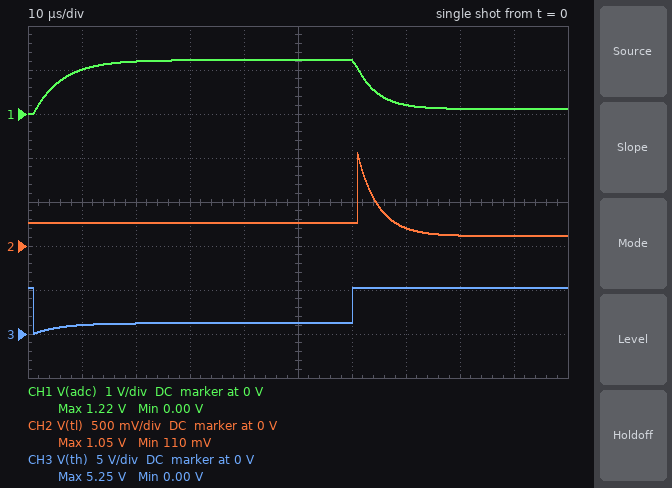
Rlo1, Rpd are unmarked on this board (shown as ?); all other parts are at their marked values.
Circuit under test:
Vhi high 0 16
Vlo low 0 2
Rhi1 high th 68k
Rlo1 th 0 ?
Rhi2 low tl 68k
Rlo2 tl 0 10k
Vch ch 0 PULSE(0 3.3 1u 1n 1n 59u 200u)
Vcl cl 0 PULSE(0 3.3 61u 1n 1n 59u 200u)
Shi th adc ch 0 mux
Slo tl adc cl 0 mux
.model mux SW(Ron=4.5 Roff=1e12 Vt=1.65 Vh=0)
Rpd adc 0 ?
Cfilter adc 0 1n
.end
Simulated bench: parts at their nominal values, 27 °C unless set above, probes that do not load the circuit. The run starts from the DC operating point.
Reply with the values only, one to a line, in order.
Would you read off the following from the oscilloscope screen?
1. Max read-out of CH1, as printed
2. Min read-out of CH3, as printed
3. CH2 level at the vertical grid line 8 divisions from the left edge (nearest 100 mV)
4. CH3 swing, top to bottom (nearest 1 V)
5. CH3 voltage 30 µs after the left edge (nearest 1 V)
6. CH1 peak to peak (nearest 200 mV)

1.22 V
0.00 V
100 mV
5 V
1 V
1.2 V
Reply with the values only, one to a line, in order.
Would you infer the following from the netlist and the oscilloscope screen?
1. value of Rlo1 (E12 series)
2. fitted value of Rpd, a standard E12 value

33 kΩ
6.8 kΩ
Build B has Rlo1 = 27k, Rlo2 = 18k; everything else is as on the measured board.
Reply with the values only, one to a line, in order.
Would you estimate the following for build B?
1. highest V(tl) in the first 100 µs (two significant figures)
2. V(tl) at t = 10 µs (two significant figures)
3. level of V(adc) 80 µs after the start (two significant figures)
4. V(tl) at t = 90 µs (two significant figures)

1.0 V
420 mV
150 mV
140 mV
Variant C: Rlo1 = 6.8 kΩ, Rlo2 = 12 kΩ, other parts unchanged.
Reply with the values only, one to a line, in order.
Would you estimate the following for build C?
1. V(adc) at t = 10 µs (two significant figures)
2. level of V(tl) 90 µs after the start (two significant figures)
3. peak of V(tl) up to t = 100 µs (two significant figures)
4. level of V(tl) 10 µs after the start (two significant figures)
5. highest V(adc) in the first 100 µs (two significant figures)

710 mV
120 mV
660 mV
300 mV
760 mV
